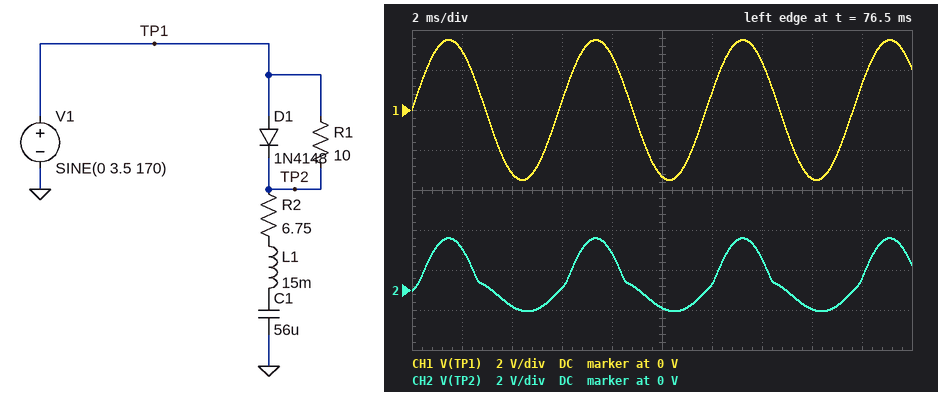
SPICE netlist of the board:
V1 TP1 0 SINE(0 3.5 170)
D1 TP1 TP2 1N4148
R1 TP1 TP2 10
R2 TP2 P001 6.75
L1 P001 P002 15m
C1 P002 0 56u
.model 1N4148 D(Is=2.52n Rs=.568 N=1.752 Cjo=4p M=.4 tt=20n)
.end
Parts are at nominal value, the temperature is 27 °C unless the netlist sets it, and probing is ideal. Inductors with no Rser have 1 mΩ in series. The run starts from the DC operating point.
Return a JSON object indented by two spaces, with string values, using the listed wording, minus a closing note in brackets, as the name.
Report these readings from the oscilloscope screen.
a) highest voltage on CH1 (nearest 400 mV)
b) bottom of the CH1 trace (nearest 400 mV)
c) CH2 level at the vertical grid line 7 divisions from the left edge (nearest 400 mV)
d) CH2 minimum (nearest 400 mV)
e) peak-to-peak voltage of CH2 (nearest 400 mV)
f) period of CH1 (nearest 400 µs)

{
  "highest voltage on CH1": "3.6 V",
  "bottom of the CH1 trace": "-3.6 V",
  "CH2 level at the vertical grid line 7 divisions from the left edge": "1.6 V",
  "CH2 minimum": "-1.2 V",
  "peak-to-peak voltage of CH2": "3.6 V",
  "period of CH1": "6.0 ms"
}
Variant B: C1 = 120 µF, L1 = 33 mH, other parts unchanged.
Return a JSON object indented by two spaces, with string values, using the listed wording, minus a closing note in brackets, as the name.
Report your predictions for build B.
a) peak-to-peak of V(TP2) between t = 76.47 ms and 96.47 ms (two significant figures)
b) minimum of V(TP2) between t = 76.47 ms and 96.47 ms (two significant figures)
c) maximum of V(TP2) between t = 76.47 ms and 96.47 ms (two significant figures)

{
  "peak-to-peak of V(TP2) between t = 76.47 ms and 96.47 ms": "6.2 V",
  "minimum of V(TP2) between t = 76.47 ms and 96.47 ms": "-3.1 V",
  "maximum of V(TP2) between t = 76.47 ms and 96.47 ms": "3.1 V"
}
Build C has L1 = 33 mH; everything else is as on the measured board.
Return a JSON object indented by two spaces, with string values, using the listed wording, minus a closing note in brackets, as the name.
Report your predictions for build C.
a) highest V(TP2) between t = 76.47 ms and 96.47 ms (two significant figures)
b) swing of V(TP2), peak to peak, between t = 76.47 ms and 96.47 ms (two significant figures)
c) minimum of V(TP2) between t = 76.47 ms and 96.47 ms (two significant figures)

{
  "highest V(TP2) between t = 76.47 ms and 96.47 ms": "2.8 V",
  "swing of V(TP2), peak to peak, between t = 76.47 ms and 96.47 ms": "5.6 V",
  "minimum of V(TP2) between t = 76.47 ms and 96.47 ms": "-2.8 V"
}
